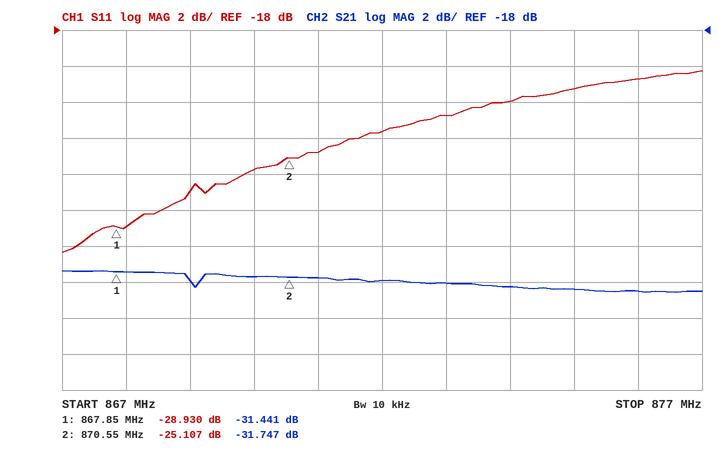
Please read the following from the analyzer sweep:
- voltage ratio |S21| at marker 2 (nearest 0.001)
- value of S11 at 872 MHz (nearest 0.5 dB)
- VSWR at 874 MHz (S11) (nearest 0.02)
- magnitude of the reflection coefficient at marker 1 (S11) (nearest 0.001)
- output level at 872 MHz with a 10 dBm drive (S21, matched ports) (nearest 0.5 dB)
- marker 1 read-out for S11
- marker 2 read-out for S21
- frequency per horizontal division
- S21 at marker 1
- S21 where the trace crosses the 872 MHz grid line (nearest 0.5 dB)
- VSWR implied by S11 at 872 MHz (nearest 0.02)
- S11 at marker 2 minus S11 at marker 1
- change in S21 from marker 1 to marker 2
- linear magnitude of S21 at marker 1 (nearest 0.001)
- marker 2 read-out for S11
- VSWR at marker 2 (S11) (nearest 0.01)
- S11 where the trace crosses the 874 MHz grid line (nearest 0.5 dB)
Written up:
0.026
-23.5 dB
1.18
0.036
-22.0 dBm
-28.930 dB
-31.747 dB
1 MHz
-31.441 dB
-32.0 dB
1.14
3.823 dB
-0.306 dB
0.027
-25.107 dB
1.12
-22.0 dB
